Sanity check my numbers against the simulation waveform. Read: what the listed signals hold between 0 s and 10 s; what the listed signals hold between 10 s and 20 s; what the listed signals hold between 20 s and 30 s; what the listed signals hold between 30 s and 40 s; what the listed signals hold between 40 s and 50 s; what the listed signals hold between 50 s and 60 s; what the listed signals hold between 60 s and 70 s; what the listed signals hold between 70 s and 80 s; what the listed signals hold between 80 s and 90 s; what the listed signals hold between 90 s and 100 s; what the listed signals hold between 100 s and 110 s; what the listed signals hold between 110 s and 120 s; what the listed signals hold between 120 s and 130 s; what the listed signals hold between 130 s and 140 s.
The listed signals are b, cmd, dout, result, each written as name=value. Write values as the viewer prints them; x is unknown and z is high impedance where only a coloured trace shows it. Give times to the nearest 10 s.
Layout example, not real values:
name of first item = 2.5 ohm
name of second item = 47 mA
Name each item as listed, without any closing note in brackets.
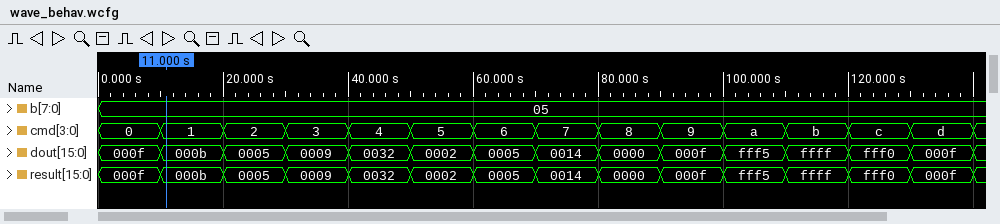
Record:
what the listed signals hold between 0 s and 10 s = b=05, cmd=0, dout=000f, result=000f
what the listed signals hold between 10 s and 20 s = b=05, cmd=1, dout=000b, result=000b
what the listed signals hold between 20 s and 30 s = b=05, cmd=2, dout=0005, result=0005
what the listed signals hold between 30 s and 40 s = b=05, cmd=3, dout=0009, result=0009
what the listed signals hold between 40 s and 50 s = b=05, cmd=4, dout=0032, result=0032
what the listed signals hold between 50 s and 60 s = b=05, cmd=5, dout=0002, result=0002
what the listed signals hold between 60 s and 70 s = b=05, cmd=6, dout=0005, result=0005
what the listed signals hold between 70 s and 80 s = b=05, cmd=7, dout=0014, result=0014
what the listed signals hold between 80 s and 90 s = b=05, cmd=8, dout=0000, result=0000
what the listed signals hold between 90 s and 100 s = b=05, cmd=9, dout=000f, result=000f
what the listed signals hold between 100 s and 110 s = b=05, cmd=a, dout=fff5, result=fff5
what the listed signals hold between 110 s and 120 s = b=05, cmd=b, dout=ffff, result=ffff
what the listed signals hold between 120 s and 130 s = b=05, cmd=c, dout=fff0, result=fff0
what the listed signals hold between 130 s and 140 s = b=05, cmd=d, dout=000f, result=000f
